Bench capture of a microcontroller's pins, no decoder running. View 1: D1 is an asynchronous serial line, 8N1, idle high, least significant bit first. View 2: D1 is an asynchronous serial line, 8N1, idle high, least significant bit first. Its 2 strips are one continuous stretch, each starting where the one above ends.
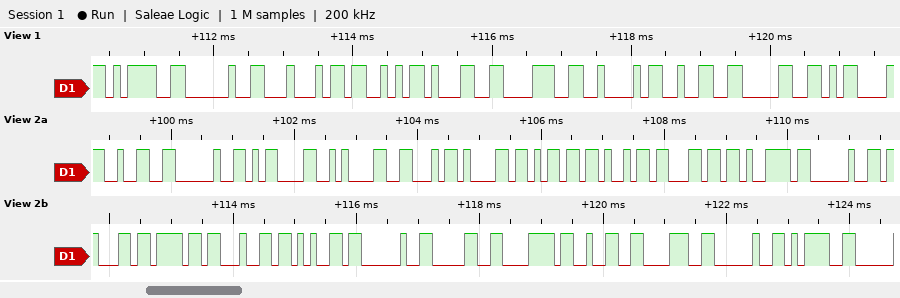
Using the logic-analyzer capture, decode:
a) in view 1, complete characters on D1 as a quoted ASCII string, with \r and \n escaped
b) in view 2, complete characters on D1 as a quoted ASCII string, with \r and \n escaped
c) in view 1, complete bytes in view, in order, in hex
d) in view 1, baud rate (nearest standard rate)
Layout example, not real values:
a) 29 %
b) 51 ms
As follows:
a) "= DS18B20\r"
b) "2 \r\nFamily code 0x28 ="
c) 3D 20 44 53 31 38 42 32 30 0D
d) 9600 baud
